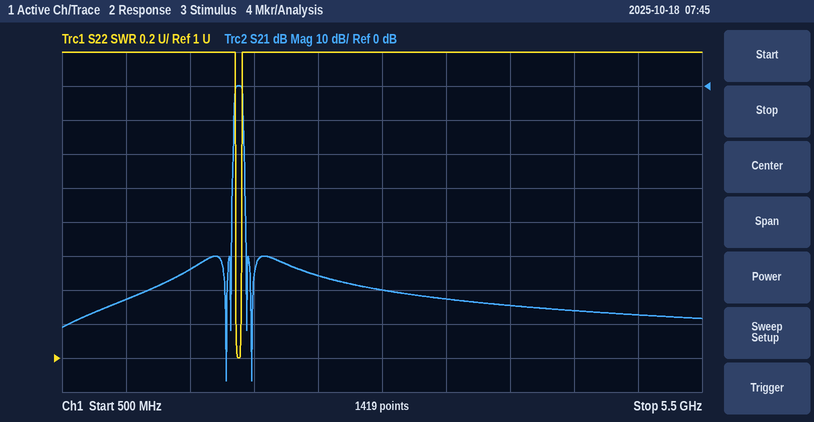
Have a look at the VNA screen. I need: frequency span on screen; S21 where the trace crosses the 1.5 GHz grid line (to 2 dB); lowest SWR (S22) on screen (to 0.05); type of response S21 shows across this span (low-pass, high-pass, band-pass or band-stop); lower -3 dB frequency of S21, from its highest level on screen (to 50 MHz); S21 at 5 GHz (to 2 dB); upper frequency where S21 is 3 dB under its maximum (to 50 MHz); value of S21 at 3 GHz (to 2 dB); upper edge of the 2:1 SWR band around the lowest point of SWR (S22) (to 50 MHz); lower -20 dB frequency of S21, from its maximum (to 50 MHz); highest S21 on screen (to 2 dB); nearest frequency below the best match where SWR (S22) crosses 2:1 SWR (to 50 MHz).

5 GHz
-54 dB
1.00
band-pass
1.85 GHz
-68 dB
1.90 GHz
-60 dB
1.90 GHz
1.85 GHz
0 dB
1.85 GHz
